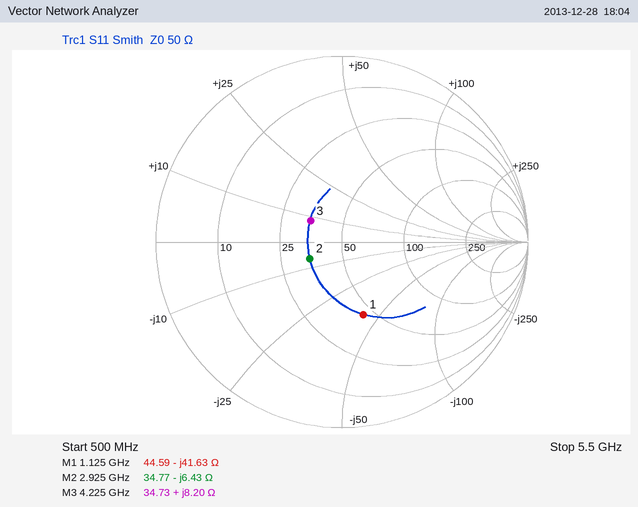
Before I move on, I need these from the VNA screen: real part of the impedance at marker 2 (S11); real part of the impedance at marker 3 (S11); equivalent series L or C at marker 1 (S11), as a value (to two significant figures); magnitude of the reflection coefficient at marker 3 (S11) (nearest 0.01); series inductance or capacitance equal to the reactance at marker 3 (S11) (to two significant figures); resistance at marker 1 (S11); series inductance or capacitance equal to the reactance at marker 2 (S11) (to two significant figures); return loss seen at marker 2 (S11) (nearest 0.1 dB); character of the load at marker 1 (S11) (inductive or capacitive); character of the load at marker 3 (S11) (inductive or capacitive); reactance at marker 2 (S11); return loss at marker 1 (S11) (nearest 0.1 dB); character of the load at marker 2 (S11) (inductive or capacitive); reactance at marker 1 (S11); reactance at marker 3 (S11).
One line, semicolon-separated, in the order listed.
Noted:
34.77 Ω; 34.73 Ω; 3.4 pF; 0.20; 310 pH; 44.59 Ω; 8.5 pF; 14.2 dB; capacitive; inductive; -6.43 Ω; 7.8 dB; capacitive; -41.63 Ω; +8.20 Ω
